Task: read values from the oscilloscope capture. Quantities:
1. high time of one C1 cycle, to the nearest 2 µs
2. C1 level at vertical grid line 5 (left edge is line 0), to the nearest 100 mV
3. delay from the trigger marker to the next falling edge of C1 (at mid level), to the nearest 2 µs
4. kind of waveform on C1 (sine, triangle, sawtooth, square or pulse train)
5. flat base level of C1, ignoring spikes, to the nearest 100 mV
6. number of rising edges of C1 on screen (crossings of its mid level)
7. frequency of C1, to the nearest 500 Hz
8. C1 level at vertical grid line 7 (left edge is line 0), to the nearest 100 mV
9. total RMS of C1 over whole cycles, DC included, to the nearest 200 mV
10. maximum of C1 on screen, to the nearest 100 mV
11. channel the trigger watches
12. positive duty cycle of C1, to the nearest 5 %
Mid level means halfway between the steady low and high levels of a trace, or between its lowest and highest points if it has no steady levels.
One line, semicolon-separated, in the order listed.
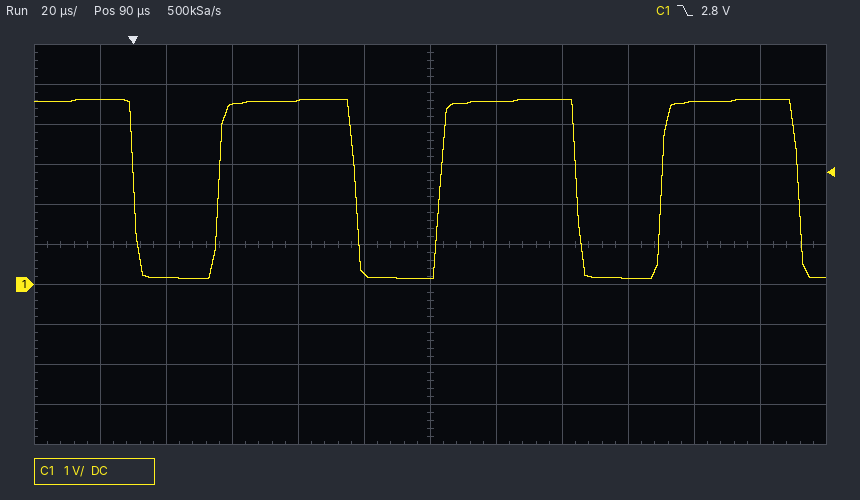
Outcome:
42 µs; 300 mV; 68 µs; pulse train; 200 mV; 3; 15.0 kHz; 4.6 V; 3.6 V; 4.6 V; C1; 60 %
